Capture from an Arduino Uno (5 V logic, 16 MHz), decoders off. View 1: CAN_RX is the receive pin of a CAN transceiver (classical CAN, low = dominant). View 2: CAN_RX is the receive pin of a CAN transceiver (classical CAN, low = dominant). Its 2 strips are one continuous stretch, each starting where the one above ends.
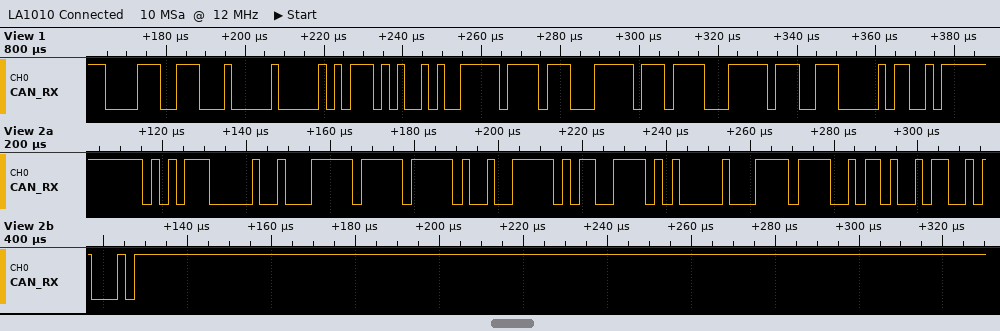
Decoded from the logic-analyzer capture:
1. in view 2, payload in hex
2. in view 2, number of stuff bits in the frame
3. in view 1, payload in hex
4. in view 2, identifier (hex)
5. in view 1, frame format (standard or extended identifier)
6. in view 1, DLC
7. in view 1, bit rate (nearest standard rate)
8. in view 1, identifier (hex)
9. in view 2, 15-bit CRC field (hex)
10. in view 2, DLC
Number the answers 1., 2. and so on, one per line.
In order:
1. FF FF 27 EC F5 00 F7 96
2. 6
3. 00 BA 94 FF B8 FF 78 FF
4. 0x570
5. standard
6. 8
7. 500 kbit/s
8. 0x0E7
9. 0x4B28
10. 8
